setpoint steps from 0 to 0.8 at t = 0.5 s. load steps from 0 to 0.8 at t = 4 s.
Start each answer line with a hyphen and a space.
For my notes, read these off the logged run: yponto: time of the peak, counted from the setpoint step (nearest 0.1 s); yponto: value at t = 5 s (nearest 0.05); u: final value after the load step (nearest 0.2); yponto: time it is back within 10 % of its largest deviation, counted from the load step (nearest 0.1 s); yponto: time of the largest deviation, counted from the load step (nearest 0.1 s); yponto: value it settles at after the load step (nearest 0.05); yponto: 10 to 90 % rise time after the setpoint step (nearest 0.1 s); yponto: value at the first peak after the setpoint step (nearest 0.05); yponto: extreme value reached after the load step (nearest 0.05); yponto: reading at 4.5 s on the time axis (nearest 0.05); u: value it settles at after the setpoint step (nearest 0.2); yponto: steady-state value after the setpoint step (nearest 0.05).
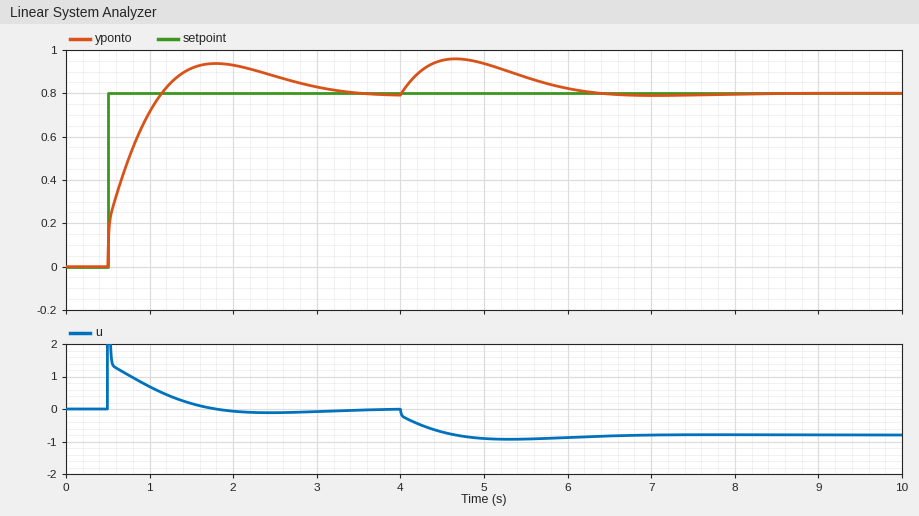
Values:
- 1.3 s
- 0.95
- -0.8
- 2.1 s
- 0.7 s
- 0.80
- 0.5 s
- 0.95
- 0.95
- 0.95
- 0.0
- 0.80
